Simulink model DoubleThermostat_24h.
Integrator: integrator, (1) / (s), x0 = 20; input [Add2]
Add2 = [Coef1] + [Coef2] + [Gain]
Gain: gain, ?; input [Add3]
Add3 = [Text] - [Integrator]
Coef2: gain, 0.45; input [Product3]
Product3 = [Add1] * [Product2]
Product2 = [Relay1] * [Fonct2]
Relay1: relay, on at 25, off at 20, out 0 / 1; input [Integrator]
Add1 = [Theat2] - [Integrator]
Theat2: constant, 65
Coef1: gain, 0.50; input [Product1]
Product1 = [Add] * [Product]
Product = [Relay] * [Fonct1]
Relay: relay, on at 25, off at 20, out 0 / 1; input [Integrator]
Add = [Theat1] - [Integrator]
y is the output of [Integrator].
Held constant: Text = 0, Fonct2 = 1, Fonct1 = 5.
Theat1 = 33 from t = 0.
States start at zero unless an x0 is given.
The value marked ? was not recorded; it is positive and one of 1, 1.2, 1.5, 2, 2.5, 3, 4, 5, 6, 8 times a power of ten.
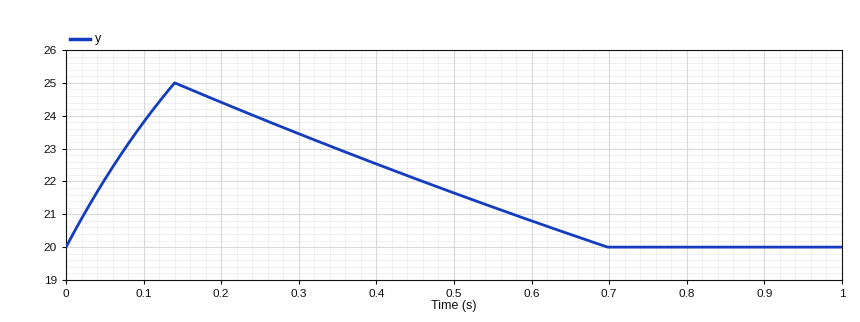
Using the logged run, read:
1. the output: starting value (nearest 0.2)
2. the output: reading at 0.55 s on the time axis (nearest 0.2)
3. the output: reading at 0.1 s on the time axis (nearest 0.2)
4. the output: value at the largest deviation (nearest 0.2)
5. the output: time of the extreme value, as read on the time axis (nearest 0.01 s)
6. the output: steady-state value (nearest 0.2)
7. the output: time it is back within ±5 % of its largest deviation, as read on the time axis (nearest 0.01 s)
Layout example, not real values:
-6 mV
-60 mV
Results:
20.0
21.2
23.8
25.0
0.14 s
20.0
0.67 s
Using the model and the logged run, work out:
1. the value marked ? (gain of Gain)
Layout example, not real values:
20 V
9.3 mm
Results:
0.4
